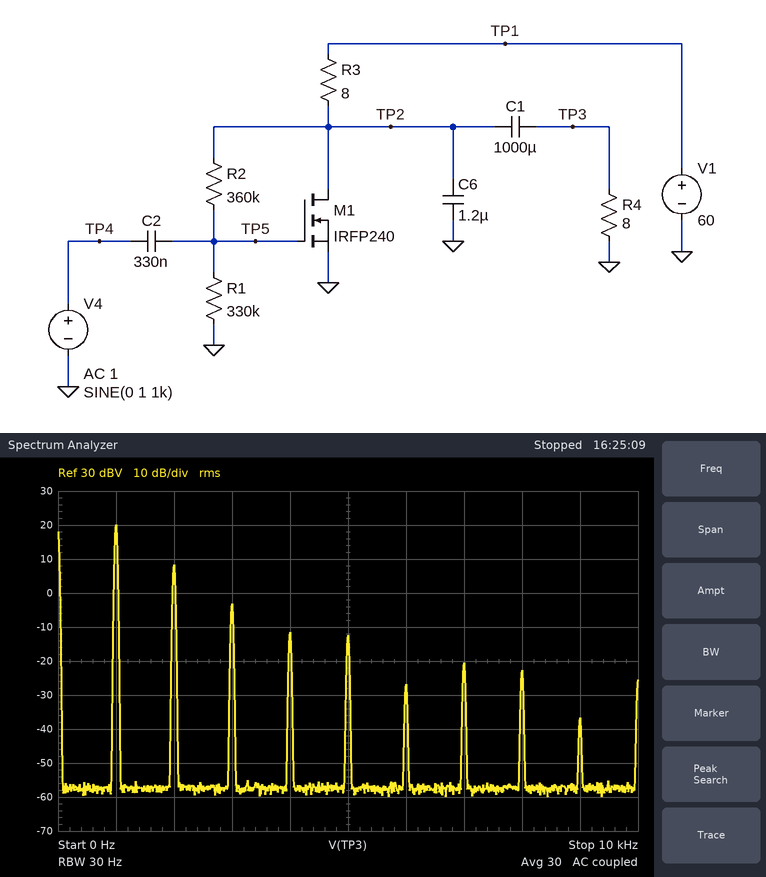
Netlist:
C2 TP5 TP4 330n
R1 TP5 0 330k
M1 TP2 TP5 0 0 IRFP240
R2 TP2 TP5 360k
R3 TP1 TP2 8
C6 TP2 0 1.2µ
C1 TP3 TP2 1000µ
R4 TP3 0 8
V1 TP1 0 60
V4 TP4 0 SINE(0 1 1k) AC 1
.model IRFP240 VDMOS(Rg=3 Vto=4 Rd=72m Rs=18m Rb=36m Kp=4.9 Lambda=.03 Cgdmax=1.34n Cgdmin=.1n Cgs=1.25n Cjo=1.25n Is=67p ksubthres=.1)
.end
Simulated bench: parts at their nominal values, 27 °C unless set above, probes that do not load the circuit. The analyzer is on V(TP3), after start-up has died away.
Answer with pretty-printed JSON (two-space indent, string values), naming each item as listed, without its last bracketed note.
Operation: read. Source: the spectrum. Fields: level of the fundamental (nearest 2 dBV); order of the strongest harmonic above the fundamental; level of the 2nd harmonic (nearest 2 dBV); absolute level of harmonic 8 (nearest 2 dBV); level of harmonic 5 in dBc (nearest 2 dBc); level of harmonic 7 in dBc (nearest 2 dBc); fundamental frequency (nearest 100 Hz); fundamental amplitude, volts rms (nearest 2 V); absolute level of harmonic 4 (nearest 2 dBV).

{
  "level of the fundamental": "20 dBV",
  "order of the strongest harmonic above the fundamental": "2",
  "level of the 2nd harmonic": "8 dBV",
  "absolute level of harmonic 8": "-22 dBV",
  "level of harmonic 5 in dBc": "-32 dBc",
  "level of harmonic 7 in dBc": "-40 dBc",
  "fundamental frequency": "1.0 kHz",
  "fundamental amplitude, volts rms": "10 V",
  "absolute level of harmonic 4": "-12 dBV"
}
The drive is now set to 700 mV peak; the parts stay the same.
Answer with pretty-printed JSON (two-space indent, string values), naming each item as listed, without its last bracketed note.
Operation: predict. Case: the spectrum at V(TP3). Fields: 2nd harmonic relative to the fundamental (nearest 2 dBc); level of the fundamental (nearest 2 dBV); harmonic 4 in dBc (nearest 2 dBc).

{
  "2nd harmonic relative to the fundamental": "-18 dBc",
  "level of the fundamental": "18 dBV",
  "harmonic 4 in dBc": "-36 dBc"
}
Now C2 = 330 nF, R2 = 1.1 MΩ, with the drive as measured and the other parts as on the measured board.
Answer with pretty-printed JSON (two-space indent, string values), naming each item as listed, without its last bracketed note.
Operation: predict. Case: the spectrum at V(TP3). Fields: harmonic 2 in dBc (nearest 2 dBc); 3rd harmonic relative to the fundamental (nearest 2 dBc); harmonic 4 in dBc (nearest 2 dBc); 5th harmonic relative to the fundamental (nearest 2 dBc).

{
  "harmonic 2 in dBc": "-30 dBc",
  "3rd harmonic relative to the fundamental": "-26 dBc",
  "harmonic 4 in dBc": "-42 dBc",
  "5th harmonic relative to the fundamental": "-56 dBc"
}
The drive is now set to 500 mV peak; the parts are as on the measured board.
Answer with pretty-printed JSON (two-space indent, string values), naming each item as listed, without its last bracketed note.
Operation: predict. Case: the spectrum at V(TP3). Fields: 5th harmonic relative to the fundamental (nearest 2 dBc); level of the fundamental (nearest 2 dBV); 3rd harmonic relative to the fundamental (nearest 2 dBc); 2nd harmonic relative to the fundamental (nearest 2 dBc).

{
  "5th harmonic relative to the fundamental": "-54 dBc",
  "level of the fundamental": "16 dBV",
  "3rd harmonic relative to the fundamental": "-38 dBc",
  "2nd harmonic relative to the fundamental": "-28 dBc"
}
